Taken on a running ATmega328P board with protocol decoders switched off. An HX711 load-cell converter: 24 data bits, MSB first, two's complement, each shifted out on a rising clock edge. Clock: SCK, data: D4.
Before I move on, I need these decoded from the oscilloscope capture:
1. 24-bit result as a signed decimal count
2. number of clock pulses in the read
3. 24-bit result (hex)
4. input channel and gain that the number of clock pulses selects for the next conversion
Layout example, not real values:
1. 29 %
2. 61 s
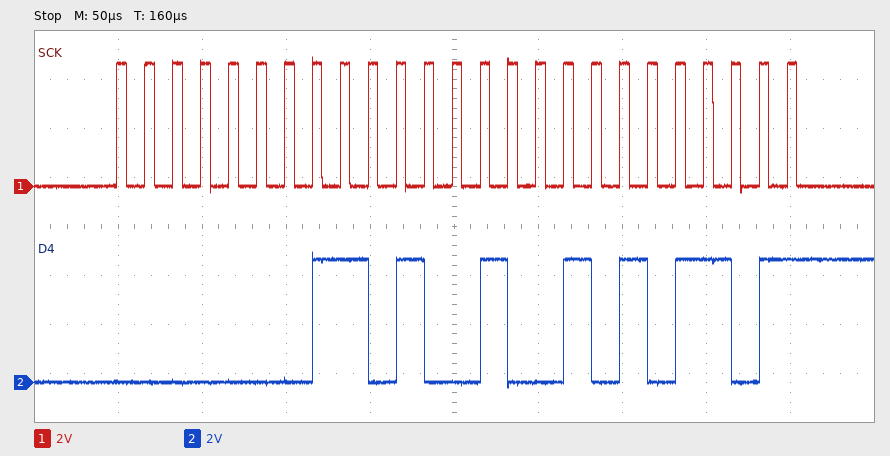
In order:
1. 107693
2. 25
3. 0x01A4AD
4. channel A, gain 128
